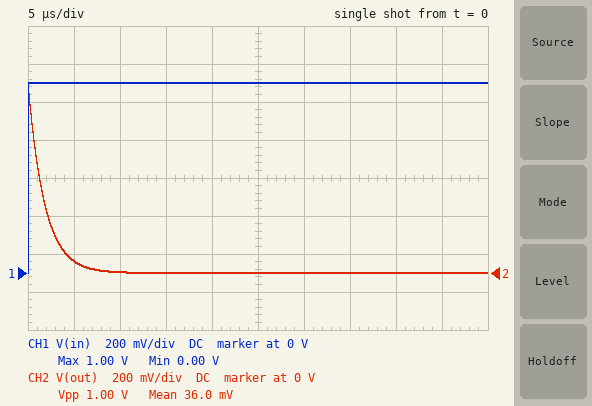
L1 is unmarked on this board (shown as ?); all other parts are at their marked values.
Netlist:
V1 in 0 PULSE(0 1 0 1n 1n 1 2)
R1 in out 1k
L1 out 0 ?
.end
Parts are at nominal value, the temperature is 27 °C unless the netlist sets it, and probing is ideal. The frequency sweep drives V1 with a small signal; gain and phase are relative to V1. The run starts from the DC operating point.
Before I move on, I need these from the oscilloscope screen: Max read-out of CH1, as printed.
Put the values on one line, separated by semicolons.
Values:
1.00 V
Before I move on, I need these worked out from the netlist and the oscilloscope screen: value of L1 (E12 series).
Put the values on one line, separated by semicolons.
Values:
1.8 mH
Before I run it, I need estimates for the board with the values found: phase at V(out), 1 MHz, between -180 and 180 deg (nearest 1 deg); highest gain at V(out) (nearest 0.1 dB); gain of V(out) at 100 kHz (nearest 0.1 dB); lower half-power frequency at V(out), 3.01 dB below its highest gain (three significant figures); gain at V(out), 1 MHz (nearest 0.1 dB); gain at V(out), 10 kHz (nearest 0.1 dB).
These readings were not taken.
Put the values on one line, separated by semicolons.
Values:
5 deg; 0 dB; -2.5 dB; 88.4 kHz; 0 dB; -19.0 dB
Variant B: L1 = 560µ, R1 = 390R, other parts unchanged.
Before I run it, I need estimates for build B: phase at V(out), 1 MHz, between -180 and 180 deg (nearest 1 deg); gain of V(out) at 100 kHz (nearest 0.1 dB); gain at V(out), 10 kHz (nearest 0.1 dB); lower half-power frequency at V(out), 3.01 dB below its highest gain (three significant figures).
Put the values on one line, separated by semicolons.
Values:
6 deg; -3.5 dB; -20.9 dB; 111 kHz
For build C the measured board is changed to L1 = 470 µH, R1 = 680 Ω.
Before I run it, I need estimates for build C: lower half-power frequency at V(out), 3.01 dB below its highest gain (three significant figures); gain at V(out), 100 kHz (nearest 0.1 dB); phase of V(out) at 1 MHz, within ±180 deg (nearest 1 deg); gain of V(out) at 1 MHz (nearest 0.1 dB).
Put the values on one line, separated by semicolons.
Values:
230 kHz; -8.0 dB; 13 deg; -0.2 dB
